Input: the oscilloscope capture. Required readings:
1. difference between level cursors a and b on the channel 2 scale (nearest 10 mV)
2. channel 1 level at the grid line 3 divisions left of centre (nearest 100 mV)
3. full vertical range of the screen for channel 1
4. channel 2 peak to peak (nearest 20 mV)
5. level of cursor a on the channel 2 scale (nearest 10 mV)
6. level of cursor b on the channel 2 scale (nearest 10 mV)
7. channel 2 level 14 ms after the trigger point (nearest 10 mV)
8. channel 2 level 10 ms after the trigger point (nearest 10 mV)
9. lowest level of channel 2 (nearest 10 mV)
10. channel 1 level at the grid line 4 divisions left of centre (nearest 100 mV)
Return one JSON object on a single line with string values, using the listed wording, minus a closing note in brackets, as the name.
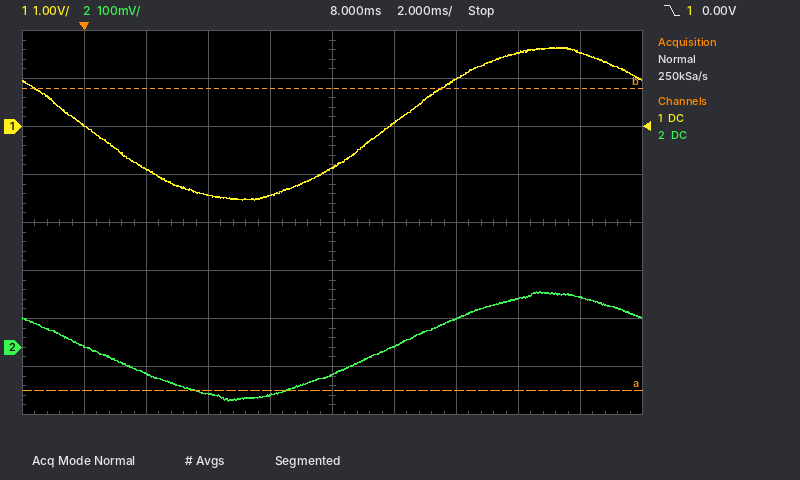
{"difference between level cursors a and b on the channel 2 scale": "630 mV", "channel 1 level at the grid line 3 divisions left of centre": "-900 mV", "full vertical range of the screen for channel 1": "8 V", "channel 2 peak to peak": "220 mV", "level of cursor a on the channel 2 scale": "-90 mV", "level of cursor b on the channel 2 scale": "540 mV", "channel 2 level 14 ms after the trigger point": "100 mV", "channel 2 level 10 ms after the trigger point": "0 mV", "lowest level of channel 2": "-110 mV", "channel 1 level at the grid line 4 divisions left of centre": "0.0 V"}
